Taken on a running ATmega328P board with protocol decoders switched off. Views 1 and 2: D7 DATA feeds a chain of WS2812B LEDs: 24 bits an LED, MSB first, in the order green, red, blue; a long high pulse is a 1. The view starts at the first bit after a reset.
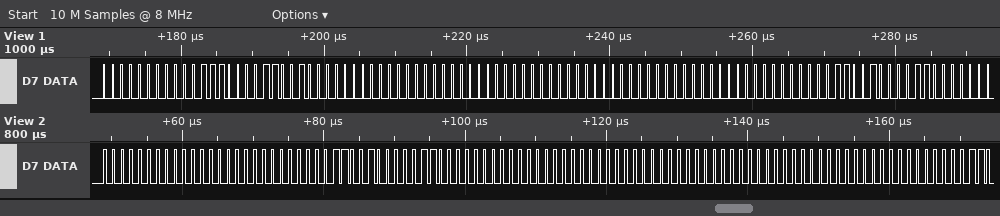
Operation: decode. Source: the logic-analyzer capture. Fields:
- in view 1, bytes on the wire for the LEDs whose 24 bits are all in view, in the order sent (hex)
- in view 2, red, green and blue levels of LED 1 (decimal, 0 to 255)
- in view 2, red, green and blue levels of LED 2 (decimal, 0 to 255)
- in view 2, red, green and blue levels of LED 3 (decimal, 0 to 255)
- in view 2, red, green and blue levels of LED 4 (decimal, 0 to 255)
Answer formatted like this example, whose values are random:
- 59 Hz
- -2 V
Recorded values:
- 00 1C 32 00 00 00 00 00 00 00 32 18
- 0, 0, 0
- 12, 50, 0
- 0, 0, 0
- 0, 0, 0
